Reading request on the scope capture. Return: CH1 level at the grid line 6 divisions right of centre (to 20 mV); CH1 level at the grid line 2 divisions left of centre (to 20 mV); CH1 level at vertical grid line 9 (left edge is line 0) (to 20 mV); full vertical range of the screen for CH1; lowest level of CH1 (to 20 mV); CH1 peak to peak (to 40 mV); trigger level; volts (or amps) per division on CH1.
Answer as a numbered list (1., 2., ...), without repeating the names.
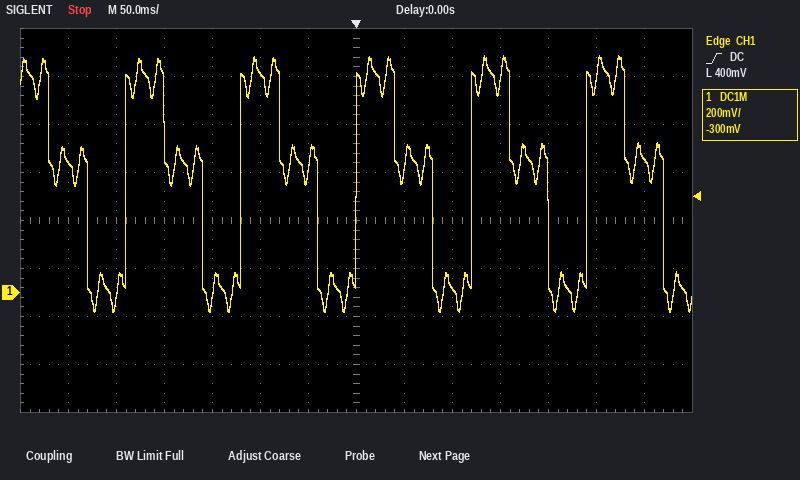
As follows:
1. 560 mV
2. 920 mV
3. 20 mV
4. 1.6 V
5. -80 mV
6. 1.08 V
7. 400 mV
8. 200 mV
